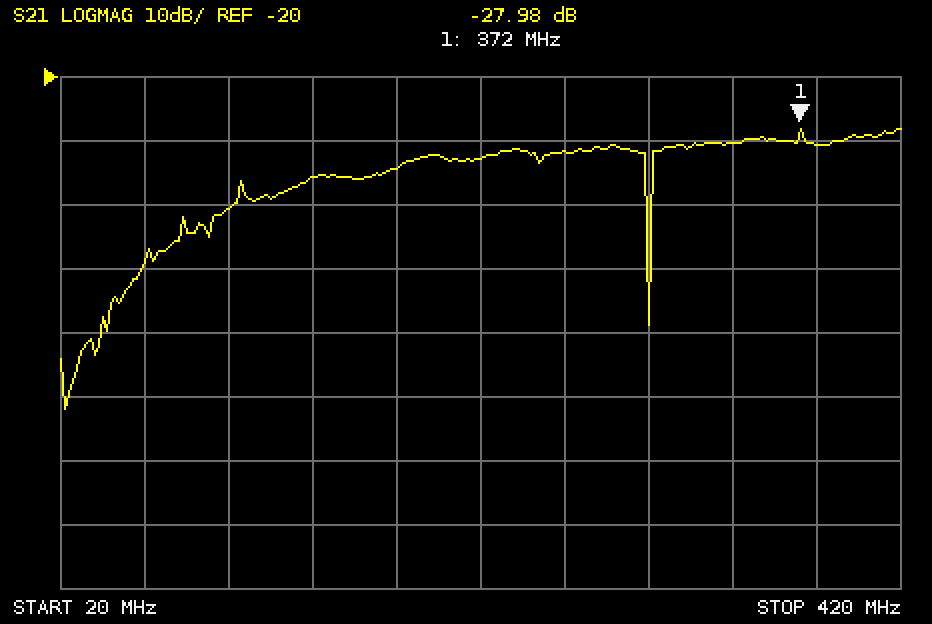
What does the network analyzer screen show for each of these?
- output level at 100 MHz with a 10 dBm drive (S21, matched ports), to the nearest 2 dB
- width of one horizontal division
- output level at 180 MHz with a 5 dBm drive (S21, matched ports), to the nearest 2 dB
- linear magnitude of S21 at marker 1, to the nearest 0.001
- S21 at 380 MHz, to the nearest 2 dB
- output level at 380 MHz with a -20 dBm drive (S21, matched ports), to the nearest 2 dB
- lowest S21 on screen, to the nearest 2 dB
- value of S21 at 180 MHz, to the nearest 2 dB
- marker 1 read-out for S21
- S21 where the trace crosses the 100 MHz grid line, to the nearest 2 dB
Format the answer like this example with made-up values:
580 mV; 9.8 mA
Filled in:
-30 dBm; 40 MHz; -30 dBm; 0.040; -30 dB; -50 dBm; -72 dB; -34 dB; -27.98 dB; -40 dB
